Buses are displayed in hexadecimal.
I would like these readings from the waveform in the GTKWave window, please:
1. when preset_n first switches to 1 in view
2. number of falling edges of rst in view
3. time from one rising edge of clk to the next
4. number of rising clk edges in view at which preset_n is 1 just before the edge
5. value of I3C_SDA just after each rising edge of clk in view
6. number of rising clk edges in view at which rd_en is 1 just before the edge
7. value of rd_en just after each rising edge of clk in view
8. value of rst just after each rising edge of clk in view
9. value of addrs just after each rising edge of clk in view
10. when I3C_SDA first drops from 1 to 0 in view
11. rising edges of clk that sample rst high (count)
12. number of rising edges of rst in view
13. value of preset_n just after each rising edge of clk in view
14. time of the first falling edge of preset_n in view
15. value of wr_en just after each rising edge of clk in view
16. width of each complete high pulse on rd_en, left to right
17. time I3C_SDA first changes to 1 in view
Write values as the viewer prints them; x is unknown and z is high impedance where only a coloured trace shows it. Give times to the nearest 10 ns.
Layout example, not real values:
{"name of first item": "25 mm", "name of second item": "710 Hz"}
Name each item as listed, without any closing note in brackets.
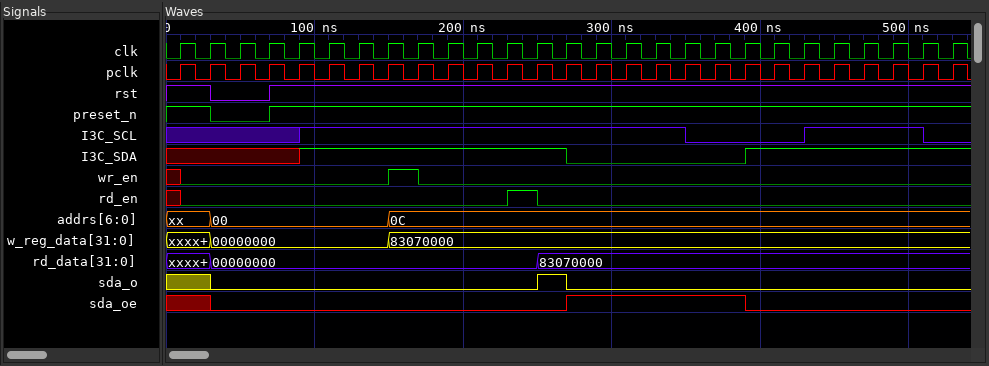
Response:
{"when preset_n first switches to 1 in view": "70 ns", "number of falling edges of rst in view": "1", "time from one rising edge of clk to the next": "20 ns", "number of rising clk edges in view at which preset_n is 1 just before the edge": "25", "value of I3C_SDA just after each rising edge of clk in view": "x x x x 1 1 1 1 1 1 1 1 1 0 0 0 0 0 0 1 1 1 1 1 1 1 1", "number of rising clk edges in view at which rd_en is 1 just before the edge": "1", "value of rd_en just after each rising edge of clk in view": "0 0 0 0 0 0 0 0 0 0 0 1 0 0 0 0 0 0 0 0 0 0 0 0 0 0 0", "value of rst just after each rising edge of clk in view": "1 0 0 1 1 1 1 1 1 1 1 1 1 1 1 1 1 1 1 1 1 1 1 1 1 1 1", "value of addrs just after each rising edge of clk in view": "xx, 00, 00, 00, 00, 00, 00, 0C, 0C, 0C, 0C, 0C, 0C, 0C, 0C, 0C, 0C, 0C, 0C, 0C, 0C, 0C, 0C, 0C, 0C, 0C, 0C", "when I3C_SDA first drops from 1 to 0 in view": "270 ns", "rising edges of clk that sample rst high": "25", "number of rising edges of rst in view": "1", "value of preset_n just after each rising edge of clk in view": "1 0 0 1 1 1 1 1 1 1 1 1 1 1 1 1 1 1 1 1 1 1 1 1 1 1 1", "time of the first falling edge of preset_n in view": "30 ns", "value of wr_en just after each rising edge of clk in view": "0 0 0 0 0 0 0 1 0 0 0 0 0 0 0 0 0 0 0 0 0 0 0 0 0 0 0", "width of each complete high pulse on rd_en, left to right": "20 ns", "time I3C_SDA first changes to 1 in view": "90 ns"}
